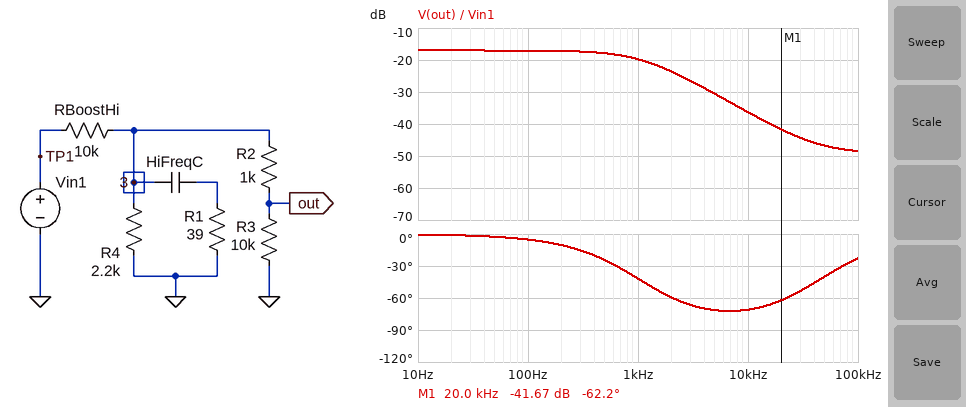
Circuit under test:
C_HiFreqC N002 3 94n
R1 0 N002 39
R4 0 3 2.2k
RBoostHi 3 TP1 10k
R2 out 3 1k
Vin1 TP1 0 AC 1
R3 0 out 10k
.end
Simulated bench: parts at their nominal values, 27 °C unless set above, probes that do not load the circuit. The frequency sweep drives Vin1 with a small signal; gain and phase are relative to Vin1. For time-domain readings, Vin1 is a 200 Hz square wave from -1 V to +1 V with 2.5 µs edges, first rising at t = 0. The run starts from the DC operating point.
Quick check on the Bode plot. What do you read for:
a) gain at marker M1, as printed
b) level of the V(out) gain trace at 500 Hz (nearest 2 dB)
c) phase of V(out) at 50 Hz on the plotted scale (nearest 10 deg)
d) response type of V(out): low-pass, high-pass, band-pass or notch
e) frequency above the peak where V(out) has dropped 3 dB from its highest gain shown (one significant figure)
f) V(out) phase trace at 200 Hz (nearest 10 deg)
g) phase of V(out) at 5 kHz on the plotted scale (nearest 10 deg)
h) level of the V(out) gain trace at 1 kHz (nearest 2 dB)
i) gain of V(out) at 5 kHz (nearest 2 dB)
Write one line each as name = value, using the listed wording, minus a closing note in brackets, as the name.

gain at marker M1, as printed = -41.67 dB
level of the V(out) gain trace at 500 Hz = -18 dB
phase of V(out) at 50 Hz on the plotted scale = 0 deg
response type of V(out): low-pass, high-pass, band-pass or notch = low-pass
frequency above the peak where V(out) has dropped 3 dB from its highest gain shown = 1 kHz
V(out) phase trace at 200 Hz = -10 deg
phase of V(out) at 5 kHz on the plotted scale = -70 deg
level of the V(out) gain trace at 1 kHz = -20 dB
gain of V(out) at 5 kHz = -30 dB
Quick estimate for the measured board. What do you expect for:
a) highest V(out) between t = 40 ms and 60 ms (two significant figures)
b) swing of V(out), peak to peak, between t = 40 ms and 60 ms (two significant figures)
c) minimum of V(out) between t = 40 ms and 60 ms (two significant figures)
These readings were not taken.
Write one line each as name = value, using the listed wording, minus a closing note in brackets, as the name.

highest V(out) between t = 40 ms and 60 ms = 140 mV
swing of V(out), peak to peak, between t = 40 ms and 60 ms = 280 mV
minimum of V(out) between t = 40 ms and 60 ms = -140 mV
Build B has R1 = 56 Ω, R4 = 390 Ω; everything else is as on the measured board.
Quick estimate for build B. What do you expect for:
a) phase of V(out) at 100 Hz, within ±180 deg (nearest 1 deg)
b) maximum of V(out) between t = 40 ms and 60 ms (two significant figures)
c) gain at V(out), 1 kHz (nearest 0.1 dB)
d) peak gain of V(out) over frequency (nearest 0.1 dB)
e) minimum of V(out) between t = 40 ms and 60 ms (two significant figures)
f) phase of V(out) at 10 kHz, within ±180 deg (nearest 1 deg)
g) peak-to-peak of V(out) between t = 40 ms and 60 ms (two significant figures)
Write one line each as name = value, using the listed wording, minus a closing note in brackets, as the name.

phase of V(out) at 100 Hz, within ±180 deg = -1 deg
maximum of V(out) between t = 40 ms and 60 ms = 33 mV
gain at V(out), 1 kHz = -29.9 dB
peak gain of V(out) over frequency = -29.6 dB
minimum of V(out) between t = 40 ms and 60 ms = -33 mV
phase of V(out) at 10 kHz, within ±180 deg = -50 deg
peak-to-peak of V(out) between t = 40 ms and 60 ms = 66 mV
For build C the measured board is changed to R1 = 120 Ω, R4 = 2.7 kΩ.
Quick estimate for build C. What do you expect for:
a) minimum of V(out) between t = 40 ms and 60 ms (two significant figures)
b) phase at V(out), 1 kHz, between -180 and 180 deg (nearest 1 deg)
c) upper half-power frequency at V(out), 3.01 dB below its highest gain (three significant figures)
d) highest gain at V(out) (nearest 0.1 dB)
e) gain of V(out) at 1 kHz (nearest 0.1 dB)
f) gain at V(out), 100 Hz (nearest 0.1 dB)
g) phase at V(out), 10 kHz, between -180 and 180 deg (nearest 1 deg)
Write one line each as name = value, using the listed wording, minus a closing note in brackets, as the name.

minimum of V(out) between t = 40 ms and 60 ms = -160 mV
phase at V(out), 1 kHz, between -180 and 180 deg = -44 deg
upper half-power frequency at V(out), 3.01 dB below its highest gain = 894 Hz
highest gain at V(out) = -15.8 dB
gain of V(out) at 1 kHz = -19.3 dB
gain at V(out), 100 Hz = -15.9 dB
phase at V(out), 10 kHz, between -180 and 180 deg = -50 deg
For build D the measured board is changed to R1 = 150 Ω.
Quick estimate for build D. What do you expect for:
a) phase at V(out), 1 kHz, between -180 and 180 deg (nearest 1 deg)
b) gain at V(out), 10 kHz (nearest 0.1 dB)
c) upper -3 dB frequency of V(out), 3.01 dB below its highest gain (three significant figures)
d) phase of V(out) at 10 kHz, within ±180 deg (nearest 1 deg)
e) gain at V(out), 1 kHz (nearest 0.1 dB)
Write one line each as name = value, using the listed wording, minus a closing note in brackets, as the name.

phase at V(out), 1 kHz, between -180 and 180 deg = -40 deg
gain at V(out), 10 kHz = -34.6 dB
upper -3 dB frequency of V(out), 3.01 dB below its highest gain = 1.00 kHz
phase of V(out) at 10 kHz, within ±180 deg = -43 deg
gain at V(out), 1 kHz = -20.0 dB
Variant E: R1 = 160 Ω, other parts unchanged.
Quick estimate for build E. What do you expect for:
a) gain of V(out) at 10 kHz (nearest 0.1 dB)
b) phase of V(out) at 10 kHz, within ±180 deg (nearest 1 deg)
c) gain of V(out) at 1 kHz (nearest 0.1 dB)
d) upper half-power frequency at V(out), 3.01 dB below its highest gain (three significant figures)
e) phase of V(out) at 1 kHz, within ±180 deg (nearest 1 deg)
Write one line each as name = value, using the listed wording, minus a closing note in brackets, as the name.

gain of V(out) at 10 kHz = -34.4 dB
phase of V(out) at 10 kHz, within ±180 deg = -41 deg
gain of V(out) at 1 kHz = -20.0 dB
upper half-power frequency at V(out), 3.01 dB below its highest gain = 999 Hz
phase of V(out) at 1 kHz, within ±180 deg = -40 deg
